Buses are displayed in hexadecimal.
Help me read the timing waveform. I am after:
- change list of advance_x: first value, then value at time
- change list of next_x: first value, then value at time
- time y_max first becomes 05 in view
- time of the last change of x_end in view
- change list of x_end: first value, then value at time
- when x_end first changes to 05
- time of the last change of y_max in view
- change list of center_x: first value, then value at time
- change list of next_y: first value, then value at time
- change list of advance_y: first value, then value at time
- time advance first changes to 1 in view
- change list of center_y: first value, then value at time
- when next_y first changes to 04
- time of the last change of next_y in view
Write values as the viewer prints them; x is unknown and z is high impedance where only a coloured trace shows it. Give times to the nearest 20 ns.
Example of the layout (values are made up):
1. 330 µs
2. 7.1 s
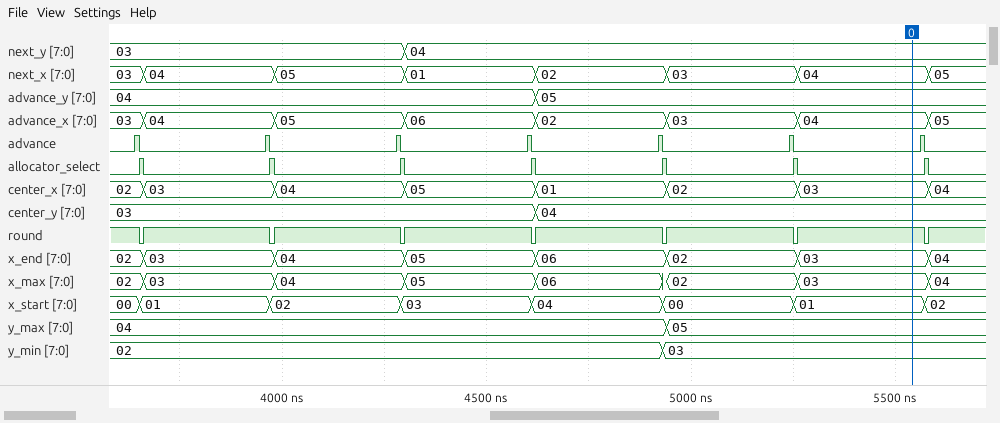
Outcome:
1. 03, 04 at 3660 ns, 05 at 3980 ns, 06 at 4300 ns, 02 at 4620 ns, 03 at 4940 ns, 04 at 5260 ns, 05 at 5580 ns
2. 03, 04 at 3660 ns, 05 at 3980 ns, 01 at 4300 ns, 02 at 4620 ns, 03 at 4940 ns, 04 at 5260 ns, 05 at 5580 ns
3. 4940 ns
4. 5580 ns
5. 02, 03 at 3660 ns, 04 at 3980 ns, 05 at 4300 ns, 06 at 4620 ns, 02 at 4940 ns, 03 at 5260 ns, 04 at 5580 ns
6. 4300 ns
7. 4940 ns
8. 02, 03 at 3660 ns, 04 at 3980 ns, 05 at 4300 ns, 01 at 4620 ns, 02 at 4940 ns, 03 at 5260 ns, 04 at 5580 ns
9. 03, 04 at 4300 ns
10. 04, 05 at 4620 ns
11. 3640 ns
12. 03, 04 at 4620 ns
13. 4300 ns
14. 4300 ns
